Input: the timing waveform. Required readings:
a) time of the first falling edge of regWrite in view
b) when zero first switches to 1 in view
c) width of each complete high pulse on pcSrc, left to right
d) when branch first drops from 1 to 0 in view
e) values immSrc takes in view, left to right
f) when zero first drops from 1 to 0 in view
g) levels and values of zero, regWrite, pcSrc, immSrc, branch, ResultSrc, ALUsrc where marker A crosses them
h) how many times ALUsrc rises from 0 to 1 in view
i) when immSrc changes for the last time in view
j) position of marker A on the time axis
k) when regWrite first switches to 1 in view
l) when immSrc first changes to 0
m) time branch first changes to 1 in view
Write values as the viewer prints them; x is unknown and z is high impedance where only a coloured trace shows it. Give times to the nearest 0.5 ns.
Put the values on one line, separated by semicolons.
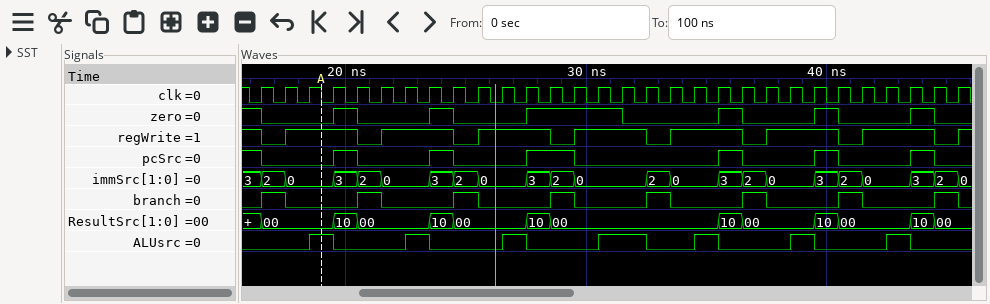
16.5 ns; 19.5 ns; 1 ns, 1 ns, 2 ns, 1 ns, 1 ns, 1 ns; 17.5 ns; 3, 2, 0, 3, 2, 0, 3, 2, 0, 3, 2, 0, 2, 0, 3, 2, 0, 3, 2, 0, 3, 2, 0; 16.5 ns; zero=0, regWrite=1, pcSrc=0, immSrc=0, branch=0, ResultSrc=00, ALUsrc=1; 7; 45.5 ns; 19 ns; 17.5 ns; 17.5 ns; 16.5 ns
